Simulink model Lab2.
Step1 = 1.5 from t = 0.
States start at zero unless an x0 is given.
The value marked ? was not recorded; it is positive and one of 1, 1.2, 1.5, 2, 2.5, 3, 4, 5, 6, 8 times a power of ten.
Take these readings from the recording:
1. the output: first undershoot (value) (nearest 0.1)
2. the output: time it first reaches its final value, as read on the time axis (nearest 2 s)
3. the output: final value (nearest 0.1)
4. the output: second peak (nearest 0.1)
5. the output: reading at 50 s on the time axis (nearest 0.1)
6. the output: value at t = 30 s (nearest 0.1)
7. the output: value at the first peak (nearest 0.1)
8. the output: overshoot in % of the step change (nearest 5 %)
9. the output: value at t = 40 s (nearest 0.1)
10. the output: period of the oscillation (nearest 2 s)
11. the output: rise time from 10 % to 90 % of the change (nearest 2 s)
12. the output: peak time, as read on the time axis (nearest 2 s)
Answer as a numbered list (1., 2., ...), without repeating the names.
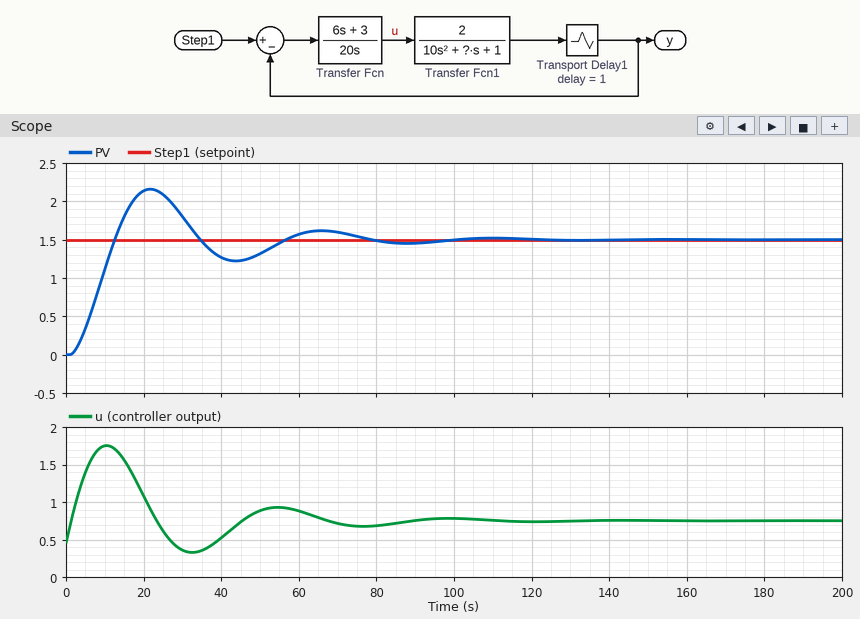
1. 1.2
2. 12 s
3. 1.5
4. 1.6
5. 1.3
6. 1.8
7. 2.2
8. 45 %
9. 1.3
10. 44 s
11. 8 s
12. 22 s
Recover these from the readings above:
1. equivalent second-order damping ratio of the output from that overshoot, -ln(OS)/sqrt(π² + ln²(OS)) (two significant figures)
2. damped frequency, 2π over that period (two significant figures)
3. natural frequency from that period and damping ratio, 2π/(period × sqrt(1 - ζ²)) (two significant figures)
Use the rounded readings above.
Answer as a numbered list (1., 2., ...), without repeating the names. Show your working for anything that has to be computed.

1. ln(0.45) = -0.799; 0.799 / sqrt(9.870 + 0.638) = 0.25
2. 2π / 44 = 0.14 rad/s
3. 2π / (44 × sqrt(1 - 0.25²)) = 0.15 rad/s
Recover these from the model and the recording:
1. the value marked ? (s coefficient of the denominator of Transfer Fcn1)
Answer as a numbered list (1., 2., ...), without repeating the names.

1. 15
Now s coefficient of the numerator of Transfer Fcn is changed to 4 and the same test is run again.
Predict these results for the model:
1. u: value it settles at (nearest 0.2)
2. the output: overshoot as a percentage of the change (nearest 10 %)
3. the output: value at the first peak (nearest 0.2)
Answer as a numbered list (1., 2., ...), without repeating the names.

1. 0.8
2. 50 %
3. 2.2
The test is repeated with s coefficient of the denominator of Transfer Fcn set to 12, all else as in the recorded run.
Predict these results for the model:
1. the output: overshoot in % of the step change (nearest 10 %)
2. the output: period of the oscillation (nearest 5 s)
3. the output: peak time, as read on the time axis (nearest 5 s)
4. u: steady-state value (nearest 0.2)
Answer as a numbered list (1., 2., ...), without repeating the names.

1. 50 %
2. 35 s
3. 15 s
4. 0.8
